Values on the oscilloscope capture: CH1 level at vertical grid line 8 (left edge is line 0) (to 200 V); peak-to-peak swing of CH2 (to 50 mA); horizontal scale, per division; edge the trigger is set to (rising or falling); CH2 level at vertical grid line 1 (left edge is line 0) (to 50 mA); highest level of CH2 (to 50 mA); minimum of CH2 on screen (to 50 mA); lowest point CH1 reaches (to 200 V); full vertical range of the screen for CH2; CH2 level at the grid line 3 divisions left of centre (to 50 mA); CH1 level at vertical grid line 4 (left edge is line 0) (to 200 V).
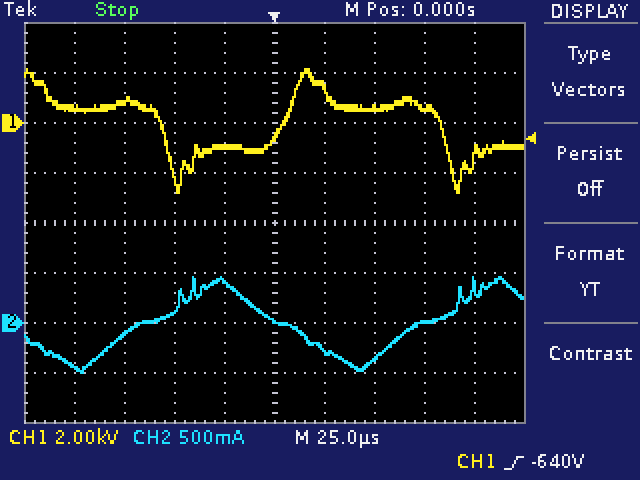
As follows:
600 V
950 mA
25 µs
rising
-450 mA
450 mA
-500 mA
-2.8 kV
4 A
-100 mA
-1.0 kV
